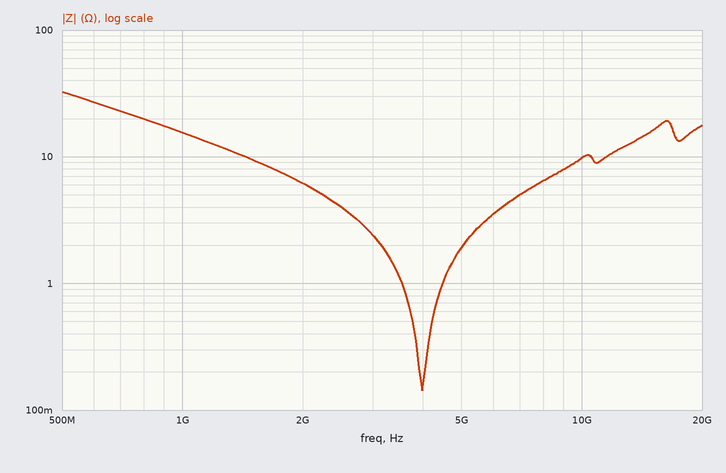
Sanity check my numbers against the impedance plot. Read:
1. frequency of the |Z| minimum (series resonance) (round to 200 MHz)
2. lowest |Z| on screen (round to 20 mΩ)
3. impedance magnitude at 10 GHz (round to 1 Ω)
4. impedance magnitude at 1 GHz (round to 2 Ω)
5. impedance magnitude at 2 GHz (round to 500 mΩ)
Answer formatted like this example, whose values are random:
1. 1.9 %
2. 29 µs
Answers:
1. 4.0 GHz
2. 140 mΩ
3. 10 Ω
4. 16 Ω
5. 6.0 Ω
